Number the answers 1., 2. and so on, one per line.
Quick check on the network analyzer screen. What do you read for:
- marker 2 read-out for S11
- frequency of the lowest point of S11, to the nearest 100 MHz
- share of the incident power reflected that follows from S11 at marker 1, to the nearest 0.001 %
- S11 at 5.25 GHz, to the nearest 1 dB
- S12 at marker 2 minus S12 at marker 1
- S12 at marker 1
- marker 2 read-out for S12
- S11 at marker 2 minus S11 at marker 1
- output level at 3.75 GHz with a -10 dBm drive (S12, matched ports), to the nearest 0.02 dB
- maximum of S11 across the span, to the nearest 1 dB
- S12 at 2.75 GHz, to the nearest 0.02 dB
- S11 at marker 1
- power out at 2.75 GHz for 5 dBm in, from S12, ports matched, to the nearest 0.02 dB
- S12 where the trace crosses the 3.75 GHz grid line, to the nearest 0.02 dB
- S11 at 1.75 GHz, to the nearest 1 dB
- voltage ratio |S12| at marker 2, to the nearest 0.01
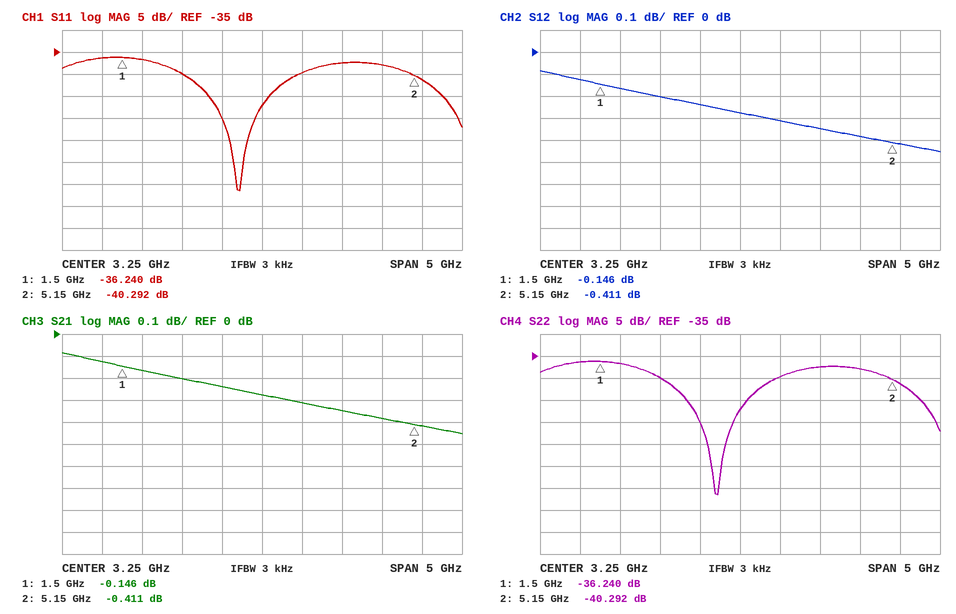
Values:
1. -40.292 dB
2. 3.0 GHz
3. 0.024 %
4. -41 dB
5. -0.265 dB
6. -0.146 dB
7. -0.411 dB
8. -4.052 dB
9. -10.32 dBm
10. -36 dB
11. -0.24 dB
12. -36.240 dB
13. 4.76 dBm
14. -0.32 dB
15. -37 dB
16. 0.95
